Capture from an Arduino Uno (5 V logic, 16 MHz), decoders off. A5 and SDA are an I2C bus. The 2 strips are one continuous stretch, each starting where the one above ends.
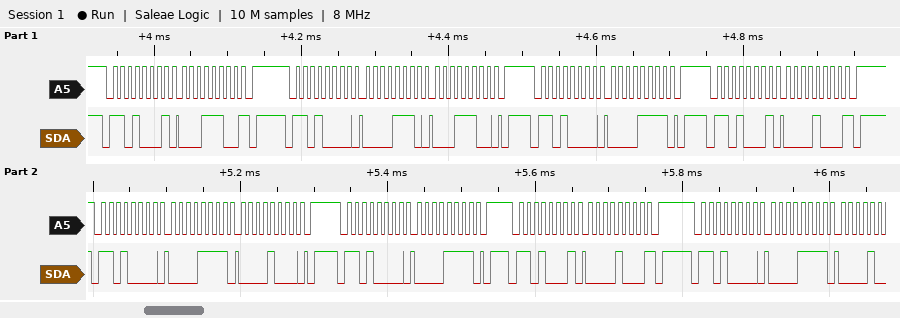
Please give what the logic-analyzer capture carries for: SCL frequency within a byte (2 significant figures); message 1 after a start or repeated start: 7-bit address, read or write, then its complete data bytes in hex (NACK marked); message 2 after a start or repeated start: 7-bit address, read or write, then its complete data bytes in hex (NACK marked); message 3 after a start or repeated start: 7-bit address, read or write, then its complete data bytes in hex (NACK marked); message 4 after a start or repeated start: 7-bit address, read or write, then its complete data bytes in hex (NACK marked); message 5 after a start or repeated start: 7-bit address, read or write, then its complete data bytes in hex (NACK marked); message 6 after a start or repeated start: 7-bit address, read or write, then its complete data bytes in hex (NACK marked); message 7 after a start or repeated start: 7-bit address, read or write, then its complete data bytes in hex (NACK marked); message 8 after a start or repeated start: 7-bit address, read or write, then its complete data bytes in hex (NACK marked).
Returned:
100 kHz
0x68 read: 1C NACK
0x68 write: 0E 1C
0x68 write: 0F
0x68 read: 08 NACK
0x68 write: 0F 08
0x68 write: 0F
0x68 read: 08 NACK
0x68 write: 0F
